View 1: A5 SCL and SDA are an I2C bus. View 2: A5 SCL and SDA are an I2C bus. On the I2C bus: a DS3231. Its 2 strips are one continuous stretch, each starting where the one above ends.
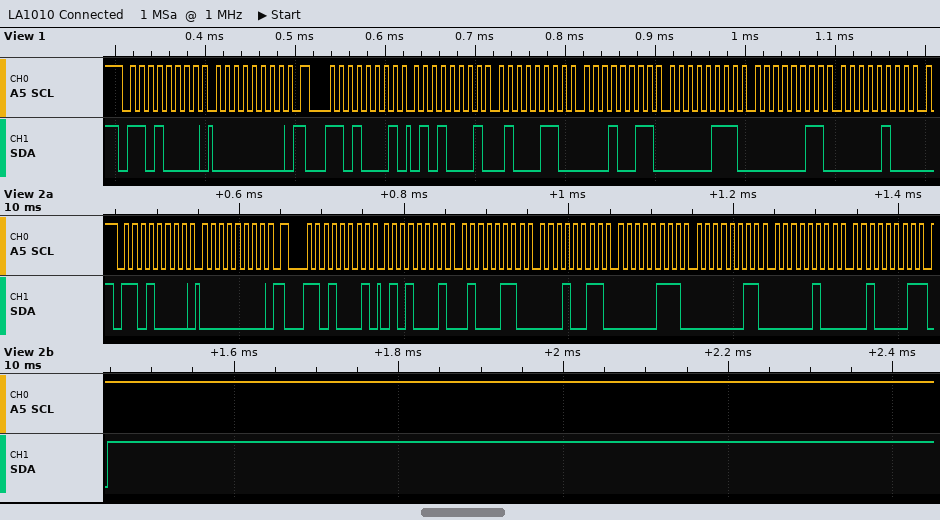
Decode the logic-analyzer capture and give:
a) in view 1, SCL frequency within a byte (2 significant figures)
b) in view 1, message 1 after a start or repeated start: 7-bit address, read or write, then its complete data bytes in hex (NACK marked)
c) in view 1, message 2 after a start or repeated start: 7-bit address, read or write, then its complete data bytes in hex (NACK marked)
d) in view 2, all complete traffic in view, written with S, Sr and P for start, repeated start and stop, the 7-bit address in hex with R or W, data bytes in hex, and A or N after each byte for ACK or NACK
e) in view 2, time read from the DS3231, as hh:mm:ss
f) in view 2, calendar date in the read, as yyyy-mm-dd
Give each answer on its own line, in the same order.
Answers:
100 kHz
0x68 write: 00
0x68 read: 51 46 13 07 03 04
S 68W A 00 A Sr 68R A 51 A 46 A 13 A 07 A 03 A 04 A 21 N P
13:46:51
2021-04-03
